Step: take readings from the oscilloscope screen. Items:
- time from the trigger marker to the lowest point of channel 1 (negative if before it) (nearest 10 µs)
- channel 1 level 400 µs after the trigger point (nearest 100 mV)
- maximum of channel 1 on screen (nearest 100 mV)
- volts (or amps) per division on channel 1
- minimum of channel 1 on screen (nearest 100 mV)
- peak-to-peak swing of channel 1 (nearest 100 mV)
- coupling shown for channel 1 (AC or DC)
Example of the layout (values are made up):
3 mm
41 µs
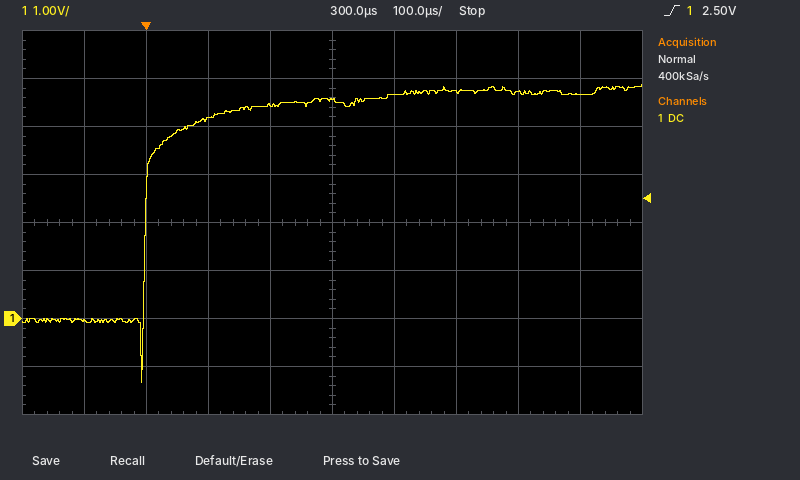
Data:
-10 µs
4.7 V
4.9 V
1 V
-1.3 V
6.2 V
DC
